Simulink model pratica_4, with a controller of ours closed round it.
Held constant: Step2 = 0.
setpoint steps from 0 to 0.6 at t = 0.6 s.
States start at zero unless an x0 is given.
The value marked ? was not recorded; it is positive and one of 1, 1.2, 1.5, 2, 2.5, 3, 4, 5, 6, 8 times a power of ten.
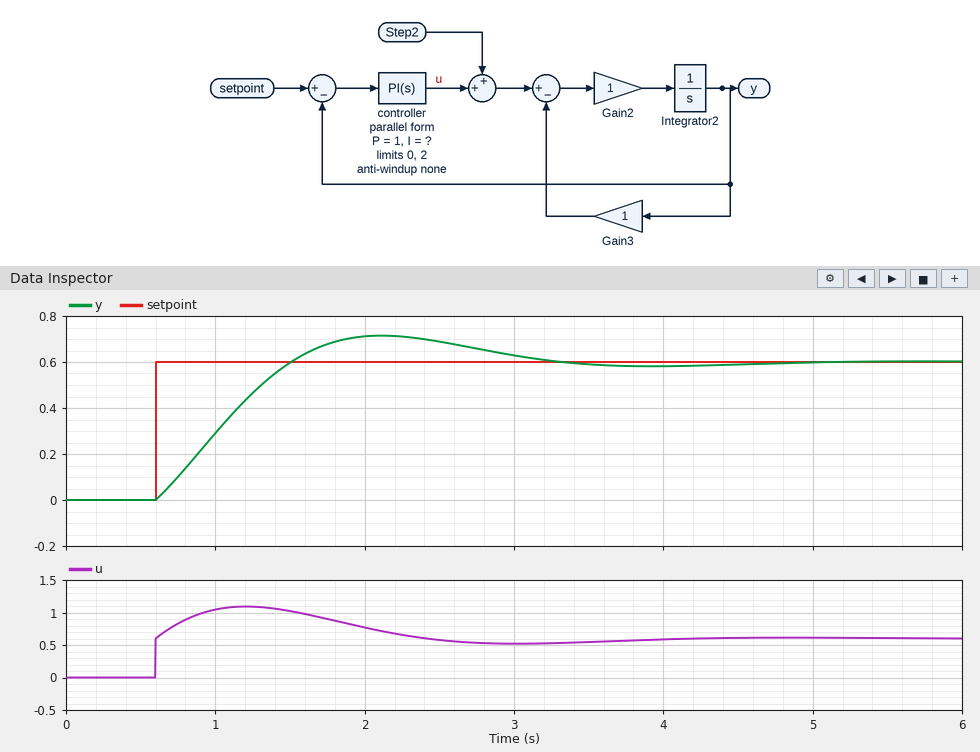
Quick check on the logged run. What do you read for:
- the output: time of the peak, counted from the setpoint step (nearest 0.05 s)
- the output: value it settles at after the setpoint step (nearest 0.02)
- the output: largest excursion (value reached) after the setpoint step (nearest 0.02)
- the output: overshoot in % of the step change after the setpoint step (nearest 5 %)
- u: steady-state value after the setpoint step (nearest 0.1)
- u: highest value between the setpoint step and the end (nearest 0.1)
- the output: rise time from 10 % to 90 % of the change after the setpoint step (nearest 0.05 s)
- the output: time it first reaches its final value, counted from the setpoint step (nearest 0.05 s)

1.50 s
0.60
0.72
20 %
0.6
1.1
0.70 s
0.90 s
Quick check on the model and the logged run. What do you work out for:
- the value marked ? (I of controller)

4
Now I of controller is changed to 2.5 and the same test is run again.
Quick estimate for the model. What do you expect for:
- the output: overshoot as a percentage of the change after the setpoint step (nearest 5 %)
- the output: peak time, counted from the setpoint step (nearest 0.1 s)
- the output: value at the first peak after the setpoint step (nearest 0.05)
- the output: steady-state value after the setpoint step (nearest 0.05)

10 %
2.0 s
0.65
0.60
